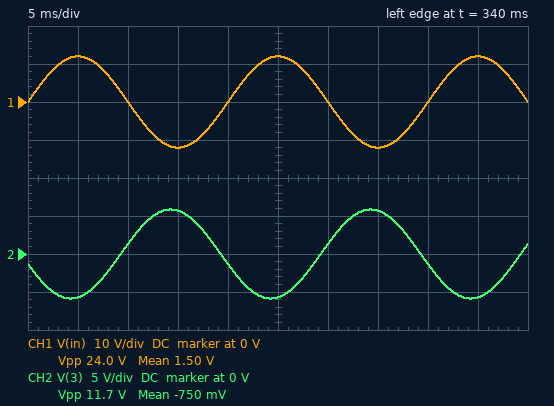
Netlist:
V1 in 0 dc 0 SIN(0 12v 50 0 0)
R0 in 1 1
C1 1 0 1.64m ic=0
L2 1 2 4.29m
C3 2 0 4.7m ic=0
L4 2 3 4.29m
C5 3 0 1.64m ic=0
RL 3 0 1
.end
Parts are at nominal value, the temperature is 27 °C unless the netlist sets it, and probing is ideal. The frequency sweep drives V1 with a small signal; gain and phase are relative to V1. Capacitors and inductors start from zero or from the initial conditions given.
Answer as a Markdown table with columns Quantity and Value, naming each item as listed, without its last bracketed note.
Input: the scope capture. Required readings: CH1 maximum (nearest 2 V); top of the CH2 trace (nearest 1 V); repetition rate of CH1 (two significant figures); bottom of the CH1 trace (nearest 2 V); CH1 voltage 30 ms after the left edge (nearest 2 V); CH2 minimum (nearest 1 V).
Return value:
| Quantity | Value |
|---|---|
| CH1 maximum | 12 V |
| top of the CH2 trace | 6 V |
| repetition rate of CH1 | 50 Hz |
| bottom of the CH1 trace | -12 V |
| CH1 voltage 30 ms after the left edge | 0 V |
| CH2 minimum | -6 V |
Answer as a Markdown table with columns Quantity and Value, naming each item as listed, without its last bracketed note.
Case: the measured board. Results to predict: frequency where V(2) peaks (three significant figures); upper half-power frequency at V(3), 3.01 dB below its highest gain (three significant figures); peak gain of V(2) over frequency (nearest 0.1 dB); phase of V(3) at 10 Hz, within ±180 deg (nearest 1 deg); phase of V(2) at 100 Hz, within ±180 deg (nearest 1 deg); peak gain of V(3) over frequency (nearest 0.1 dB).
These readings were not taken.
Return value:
| Quantity | Value |
|---|---|
| frequency where V(2) peaks | 54.6 Hz |
| upper half-power frequency at V(3), 3.01 dB below its highest gain | 63.8 Hz |
| peak gain of V(2) over frequency | -3.2 dB |
| phase of V(3) at 10 Hz, within ±180 deg | -30 deg |
| phase of V(2) at 100 Hz, within ±180 deg | 152 deg |
| peak gain of V(3) over frequency | -6.0 dB |
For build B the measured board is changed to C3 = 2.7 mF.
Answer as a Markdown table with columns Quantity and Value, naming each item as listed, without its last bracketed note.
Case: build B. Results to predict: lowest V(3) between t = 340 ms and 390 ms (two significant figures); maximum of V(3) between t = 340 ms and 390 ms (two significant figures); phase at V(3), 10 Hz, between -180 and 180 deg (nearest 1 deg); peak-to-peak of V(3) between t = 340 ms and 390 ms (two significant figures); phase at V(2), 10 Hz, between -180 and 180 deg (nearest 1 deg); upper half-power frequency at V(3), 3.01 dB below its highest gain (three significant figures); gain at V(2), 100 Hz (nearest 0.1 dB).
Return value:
| Quantity | Value |
|---|---|
| lowest V(3) between t = 340 ms and 390 ms | -5.6 V |
| maximum of V(3) between t = 340 ms and 390 ms | 5.6 V |
| phase at V(3), 10 Hz, between -180 and 180 deg | -26 deg |
| peak-to-peak of V(3) between t = 340 ms and 390 ms | 11 V |
| phase at V(2), 10 Hz, between -180 and 180 deg | -11 deg |
| upper half-power frequency at V(3), 3.01 dB below its highest gain | 82.2 Hz |
| gain at V(2), 100 Hz | -8.8 dB |
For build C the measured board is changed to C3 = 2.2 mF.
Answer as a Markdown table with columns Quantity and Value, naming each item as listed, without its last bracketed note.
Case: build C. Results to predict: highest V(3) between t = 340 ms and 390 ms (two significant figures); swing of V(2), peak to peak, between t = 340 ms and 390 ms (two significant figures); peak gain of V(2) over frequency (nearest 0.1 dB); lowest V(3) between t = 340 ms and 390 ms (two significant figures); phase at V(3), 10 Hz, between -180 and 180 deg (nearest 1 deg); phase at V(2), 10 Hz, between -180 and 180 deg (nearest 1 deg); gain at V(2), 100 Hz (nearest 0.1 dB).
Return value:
| Quantity | Value |
|---|---|
| highest V(3) between t = 340 ms and 390 ms | 5.3 V |
| swing of V(2), peak to peak, between t = 340 ms and 390 ms | 15 V |
| peak gain of V(2) over frequency | 1.2 dB |
| lowest V(3) between t = 340 ms and 390 ms | -5.3 V |
| phase at V(3), 10 Hz, between -180 and 180 deg | -25 deg |
| phase at V(2), 10 Hz, between -180 and 180 deg | -10 deg |
| gain at V(2), 100 Hz | -5.0 dB |
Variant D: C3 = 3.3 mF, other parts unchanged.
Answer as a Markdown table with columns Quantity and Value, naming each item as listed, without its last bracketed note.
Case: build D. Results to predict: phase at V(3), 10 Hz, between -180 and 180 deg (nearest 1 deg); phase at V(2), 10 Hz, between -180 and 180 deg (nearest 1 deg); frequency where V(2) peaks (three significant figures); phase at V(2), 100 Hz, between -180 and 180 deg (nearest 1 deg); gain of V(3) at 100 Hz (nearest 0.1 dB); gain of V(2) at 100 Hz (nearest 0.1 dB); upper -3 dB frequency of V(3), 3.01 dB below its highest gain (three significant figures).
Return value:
| Quantity | Value |
|---|---|
| phase at V(3), 10 Hz, between -180 and 180 deg | -27 deg |
| phase at V(2), 10 Hz, between -180 and 180 deg | -12 deg |
| frequency where V(2) peaks | 66.9 Hz |
| phase at V(2), 100 Hz, between -180 and 180 deg | 156 deg |
| gain of V(3) at 100 Hz | -22.1 dB |
| gain of V(2) at 100 Hz | -11.9 dB |
| upper -3 dB frequency of V(3), 3.01 dB below its highest gain | 75.3 Hz |
